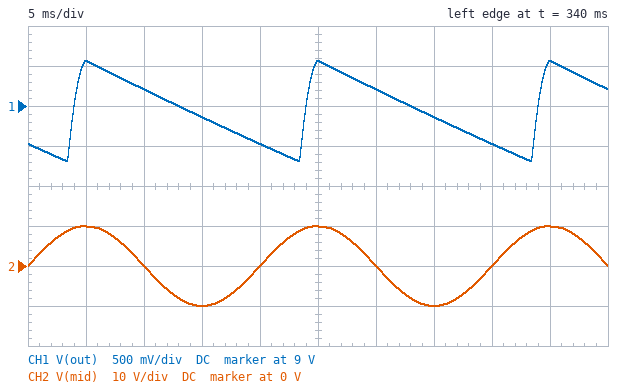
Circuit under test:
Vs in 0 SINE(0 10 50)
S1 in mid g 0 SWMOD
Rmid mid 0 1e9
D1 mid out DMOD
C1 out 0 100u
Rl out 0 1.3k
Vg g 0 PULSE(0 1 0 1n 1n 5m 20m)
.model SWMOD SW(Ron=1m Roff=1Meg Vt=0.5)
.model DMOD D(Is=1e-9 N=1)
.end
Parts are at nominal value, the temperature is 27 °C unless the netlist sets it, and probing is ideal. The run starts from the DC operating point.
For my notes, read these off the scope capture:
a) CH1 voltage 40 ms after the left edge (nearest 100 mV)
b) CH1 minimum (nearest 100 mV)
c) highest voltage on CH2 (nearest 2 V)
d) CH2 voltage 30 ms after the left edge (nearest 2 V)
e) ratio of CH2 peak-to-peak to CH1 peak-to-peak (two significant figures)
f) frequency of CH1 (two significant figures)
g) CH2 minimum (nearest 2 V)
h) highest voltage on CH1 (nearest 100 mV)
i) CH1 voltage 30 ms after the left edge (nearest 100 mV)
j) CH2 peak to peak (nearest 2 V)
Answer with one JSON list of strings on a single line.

["8.5 V", "8.3 V", "10 V", "0 V", "16", "50 Hz", "-10 V", "9.6 V", "9.2 V", "20 V"]
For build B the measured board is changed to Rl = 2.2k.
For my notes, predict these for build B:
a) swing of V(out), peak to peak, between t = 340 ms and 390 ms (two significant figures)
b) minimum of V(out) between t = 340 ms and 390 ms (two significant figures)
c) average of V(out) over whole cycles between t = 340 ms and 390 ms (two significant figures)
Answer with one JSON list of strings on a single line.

["780 mV", "8.8 V", "9.2 V"]
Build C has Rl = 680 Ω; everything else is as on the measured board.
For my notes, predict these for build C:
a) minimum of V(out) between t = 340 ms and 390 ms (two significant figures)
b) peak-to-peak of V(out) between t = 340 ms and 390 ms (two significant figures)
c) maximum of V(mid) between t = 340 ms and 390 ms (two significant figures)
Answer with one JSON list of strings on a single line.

["7.4 V", "2.2 V", "10 V"]
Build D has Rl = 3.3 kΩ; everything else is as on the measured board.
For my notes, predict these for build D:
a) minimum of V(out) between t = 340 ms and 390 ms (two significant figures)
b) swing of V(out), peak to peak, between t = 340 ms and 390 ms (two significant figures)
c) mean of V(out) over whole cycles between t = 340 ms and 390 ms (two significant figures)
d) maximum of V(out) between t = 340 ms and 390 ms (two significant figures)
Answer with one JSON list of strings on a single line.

["9.0 V", "530 mV", "9.3 V", "9.6 V"]
